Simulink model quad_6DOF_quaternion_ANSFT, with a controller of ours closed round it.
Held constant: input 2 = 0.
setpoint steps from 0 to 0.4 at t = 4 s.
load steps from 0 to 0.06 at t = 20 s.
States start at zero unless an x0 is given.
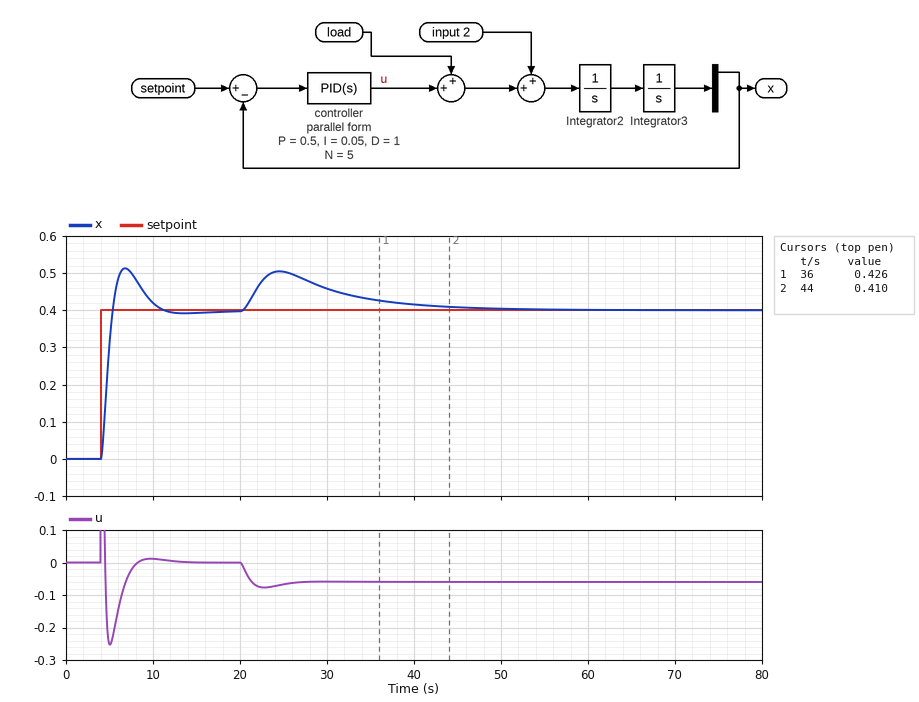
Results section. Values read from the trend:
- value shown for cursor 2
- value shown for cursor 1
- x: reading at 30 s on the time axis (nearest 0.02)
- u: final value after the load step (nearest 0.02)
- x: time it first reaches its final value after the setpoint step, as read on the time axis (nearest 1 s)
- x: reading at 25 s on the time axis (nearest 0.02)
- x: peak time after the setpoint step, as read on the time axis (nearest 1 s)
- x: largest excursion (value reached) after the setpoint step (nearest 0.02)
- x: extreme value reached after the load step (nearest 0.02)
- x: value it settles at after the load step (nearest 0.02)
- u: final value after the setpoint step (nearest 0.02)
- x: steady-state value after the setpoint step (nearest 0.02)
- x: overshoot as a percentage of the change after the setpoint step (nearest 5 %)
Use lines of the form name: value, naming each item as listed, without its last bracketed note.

value shown for cursor 2: 0.410
value shown for cursor 1: 0.426
x: reading at 30 s on the time axis: 0.46
u: final value after the load step: -0.06
x: time it first reaches its final value after the setpoint step, as read on the time axis: 5 s
x: reading at 25 s on the time axis: 0.50
x: peak time after the setpoint step, as read on the time axis: 7 s
x: largest excursion (value reached) after the setpoint step: 0.52
x: extreme value reached after the load step: 0.50
x: value it settles at after the load step: 0.40
u: final value after the setpoint step: 0.00
x: steady-state value after the setpoint step: 0.40
x: overshoot as a percentage of the change after the setpoint step: 30 %
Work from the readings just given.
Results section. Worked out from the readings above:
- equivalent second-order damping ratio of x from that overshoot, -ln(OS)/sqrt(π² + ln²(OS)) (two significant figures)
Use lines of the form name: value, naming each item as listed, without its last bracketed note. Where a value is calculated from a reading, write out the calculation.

equivalent second-order damping ratio of x from that overshoot, -ln(OS)/sqrt(π² + ln²(OS)): ln(0.3) = -1.204; 1.204 / sqrt(9.870 + 1.450) = 0.36
